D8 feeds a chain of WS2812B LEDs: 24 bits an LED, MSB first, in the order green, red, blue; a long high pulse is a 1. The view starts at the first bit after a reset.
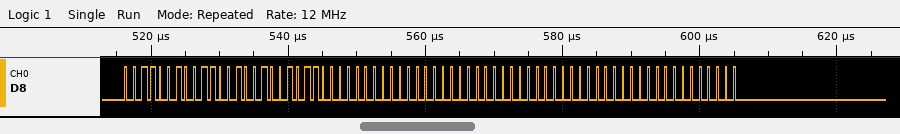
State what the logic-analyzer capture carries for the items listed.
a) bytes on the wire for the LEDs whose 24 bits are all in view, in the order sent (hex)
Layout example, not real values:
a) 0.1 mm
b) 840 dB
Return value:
a) 32 64 96 00 00 00 00 00 00
